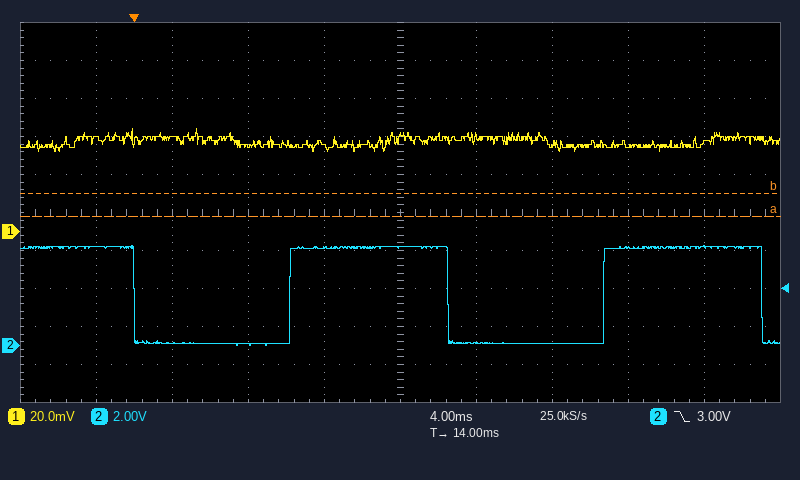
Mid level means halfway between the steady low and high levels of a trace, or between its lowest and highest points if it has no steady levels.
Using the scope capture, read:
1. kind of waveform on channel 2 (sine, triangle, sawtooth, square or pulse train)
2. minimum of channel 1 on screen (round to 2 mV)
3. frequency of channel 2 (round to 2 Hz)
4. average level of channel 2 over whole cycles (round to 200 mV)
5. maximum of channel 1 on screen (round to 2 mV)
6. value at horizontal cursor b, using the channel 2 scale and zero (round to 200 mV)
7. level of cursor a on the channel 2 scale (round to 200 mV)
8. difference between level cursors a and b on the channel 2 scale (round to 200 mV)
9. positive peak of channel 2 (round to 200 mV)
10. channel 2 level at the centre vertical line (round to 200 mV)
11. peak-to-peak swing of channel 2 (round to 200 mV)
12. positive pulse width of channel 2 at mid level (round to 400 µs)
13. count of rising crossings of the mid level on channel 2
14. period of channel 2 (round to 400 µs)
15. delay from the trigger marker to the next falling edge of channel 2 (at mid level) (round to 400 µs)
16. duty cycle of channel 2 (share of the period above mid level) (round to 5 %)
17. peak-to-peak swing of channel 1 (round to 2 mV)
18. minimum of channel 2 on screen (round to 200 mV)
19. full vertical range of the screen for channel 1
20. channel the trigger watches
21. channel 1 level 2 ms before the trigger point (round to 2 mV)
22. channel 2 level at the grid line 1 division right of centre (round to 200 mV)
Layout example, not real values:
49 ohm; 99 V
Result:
square; 42 mV; 60 Hz; 2.6 V; 54 mV; 8.0 V; 6.8 V; 1.2 V; 5.2 V; 5.2 V; 5.2 V; 8.4 ms; 2; 16.4 ms; 16.4 ms; 50 %; 12 mV; 0.0 V; 200 mV; channel 2; 48 mV; 200 mV
